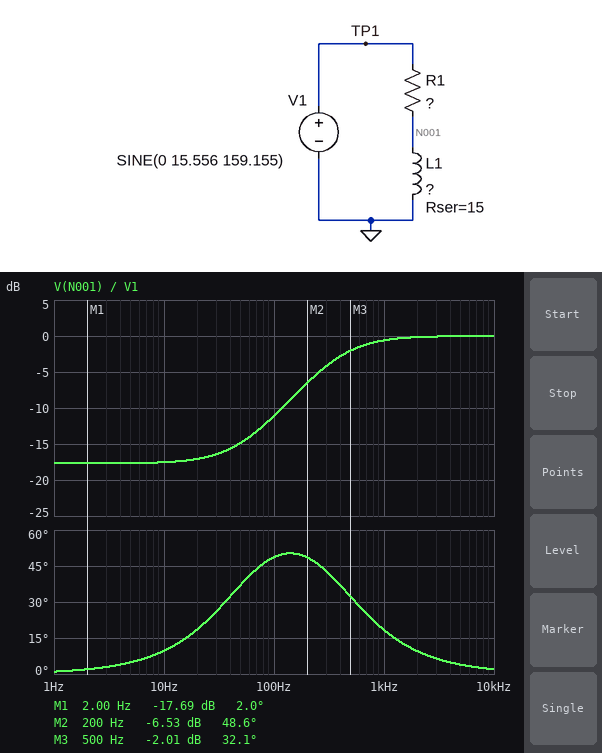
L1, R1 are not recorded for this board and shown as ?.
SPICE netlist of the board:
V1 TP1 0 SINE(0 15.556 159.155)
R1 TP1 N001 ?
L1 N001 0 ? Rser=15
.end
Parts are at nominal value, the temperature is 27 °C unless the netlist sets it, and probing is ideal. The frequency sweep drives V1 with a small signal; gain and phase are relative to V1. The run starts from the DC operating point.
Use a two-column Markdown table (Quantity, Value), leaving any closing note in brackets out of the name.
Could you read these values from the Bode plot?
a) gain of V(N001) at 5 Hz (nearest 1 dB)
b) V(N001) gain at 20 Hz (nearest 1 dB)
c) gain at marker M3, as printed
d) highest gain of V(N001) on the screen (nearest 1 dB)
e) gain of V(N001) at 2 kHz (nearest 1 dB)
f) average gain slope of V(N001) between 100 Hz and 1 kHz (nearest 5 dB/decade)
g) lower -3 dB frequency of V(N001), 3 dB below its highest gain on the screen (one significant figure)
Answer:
| Quantity | Value |
|---|---|
| gain of V(N001) at 5 Hz | -18 dB |
| V(N001) gain at 20 Hz | -17 dB |
| gain at marker M3, as printed | -2.01 dB |
| highest gain of V(N001) on the screen | 0 dB |
| gain of V(N001) at 2 kHz | 0 dB |
| average gain slope of V(N001) between 100 Hz and 1 kHz | 10 dB/decade |
| lower -3 dB frequency of V(N001), 3 dB below its highest gain on the screen | 400 Hz |
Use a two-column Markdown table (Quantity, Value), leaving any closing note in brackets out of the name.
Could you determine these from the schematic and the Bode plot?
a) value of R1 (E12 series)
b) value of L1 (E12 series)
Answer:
| Quantity | Value |
|---|---|
| value of R1 | 100 Ω |
| value of L1 | 47 mH |
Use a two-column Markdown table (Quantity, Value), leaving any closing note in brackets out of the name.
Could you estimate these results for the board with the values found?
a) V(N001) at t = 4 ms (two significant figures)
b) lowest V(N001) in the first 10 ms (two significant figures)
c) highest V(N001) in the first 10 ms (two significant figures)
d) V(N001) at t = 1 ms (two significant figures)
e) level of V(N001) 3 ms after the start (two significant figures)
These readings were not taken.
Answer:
| Quantity | Value |
|---|---|
| V(N001) at t = 4 ms | -6.1 V |
| lowest V(N001) in the first 10 ms | -6.2 V |
| highest V(N001) in the first 10 ms | 6.2 V |
| V(N001) at t = 1 ms | 5.5 V |
| level of V(N001) 3 ms after the start | -4.1 V |
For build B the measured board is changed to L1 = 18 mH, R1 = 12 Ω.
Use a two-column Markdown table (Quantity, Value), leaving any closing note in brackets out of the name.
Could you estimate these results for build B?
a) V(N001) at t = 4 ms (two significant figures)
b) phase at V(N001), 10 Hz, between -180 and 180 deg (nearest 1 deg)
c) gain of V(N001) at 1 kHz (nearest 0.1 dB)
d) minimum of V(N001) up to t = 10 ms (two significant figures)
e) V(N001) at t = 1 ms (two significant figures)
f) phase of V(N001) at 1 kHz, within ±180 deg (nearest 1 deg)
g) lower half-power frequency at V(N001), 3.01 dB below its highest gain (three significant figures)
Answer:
| Quantity | Value |
|---|---|
| V(N001) at t = 4 ms | -10 V |
| phase at V(N001), 10 Hz, between -180 and 180 deg | 2 deg |
| gain of V(N001) at 1 kHz | -0.2 dB |
| minimum of V(N001) up to t = 10 ms | -11 V |
| V(N001) at t = 1 ms | 10 V |
| phase of V(N001) at 1 kHz, within ±180 deg | 6 deg |
| lower half-power frequency at V(N001), 3.01 dB below its highest gain | 148 Hz |
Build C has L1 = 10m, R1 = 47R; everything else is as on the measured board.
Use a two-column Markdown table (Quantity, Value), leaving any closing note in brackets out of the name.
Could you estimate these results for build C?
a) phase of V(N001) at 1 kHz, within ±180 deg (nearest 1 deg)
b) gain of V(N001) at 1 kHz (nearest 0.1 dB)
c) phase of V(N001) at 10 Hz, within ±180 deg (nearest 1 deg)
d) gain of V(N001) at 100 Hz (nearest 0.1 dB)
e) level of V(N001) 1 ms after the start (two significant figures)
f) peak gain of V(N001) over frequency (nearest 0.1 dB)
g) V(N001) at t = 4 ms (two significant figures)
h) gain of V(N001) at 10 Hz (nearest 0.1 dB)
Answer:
| Quantity | Value |
|---|---|
| phase of V(N001) at 1 kHz, within ±180 deg | 31 deg |
| gain of V(N001) at 1 kHz | -2.7 dB |
| phase of V(N001) at 10 Hz, within ±180 deg | 2 deg |
| gain of V(N001) at 100 Hz | -11.7 dB |
| level of V(N001) 1 ms after the start | 4.4 V |
| peak gain of V(N001) over frequency | 0 dB |
| V(N001) at t = 4 ms | -4.3 V |
| gain of V(N001) at 10 Hz | -12.3 dB |
